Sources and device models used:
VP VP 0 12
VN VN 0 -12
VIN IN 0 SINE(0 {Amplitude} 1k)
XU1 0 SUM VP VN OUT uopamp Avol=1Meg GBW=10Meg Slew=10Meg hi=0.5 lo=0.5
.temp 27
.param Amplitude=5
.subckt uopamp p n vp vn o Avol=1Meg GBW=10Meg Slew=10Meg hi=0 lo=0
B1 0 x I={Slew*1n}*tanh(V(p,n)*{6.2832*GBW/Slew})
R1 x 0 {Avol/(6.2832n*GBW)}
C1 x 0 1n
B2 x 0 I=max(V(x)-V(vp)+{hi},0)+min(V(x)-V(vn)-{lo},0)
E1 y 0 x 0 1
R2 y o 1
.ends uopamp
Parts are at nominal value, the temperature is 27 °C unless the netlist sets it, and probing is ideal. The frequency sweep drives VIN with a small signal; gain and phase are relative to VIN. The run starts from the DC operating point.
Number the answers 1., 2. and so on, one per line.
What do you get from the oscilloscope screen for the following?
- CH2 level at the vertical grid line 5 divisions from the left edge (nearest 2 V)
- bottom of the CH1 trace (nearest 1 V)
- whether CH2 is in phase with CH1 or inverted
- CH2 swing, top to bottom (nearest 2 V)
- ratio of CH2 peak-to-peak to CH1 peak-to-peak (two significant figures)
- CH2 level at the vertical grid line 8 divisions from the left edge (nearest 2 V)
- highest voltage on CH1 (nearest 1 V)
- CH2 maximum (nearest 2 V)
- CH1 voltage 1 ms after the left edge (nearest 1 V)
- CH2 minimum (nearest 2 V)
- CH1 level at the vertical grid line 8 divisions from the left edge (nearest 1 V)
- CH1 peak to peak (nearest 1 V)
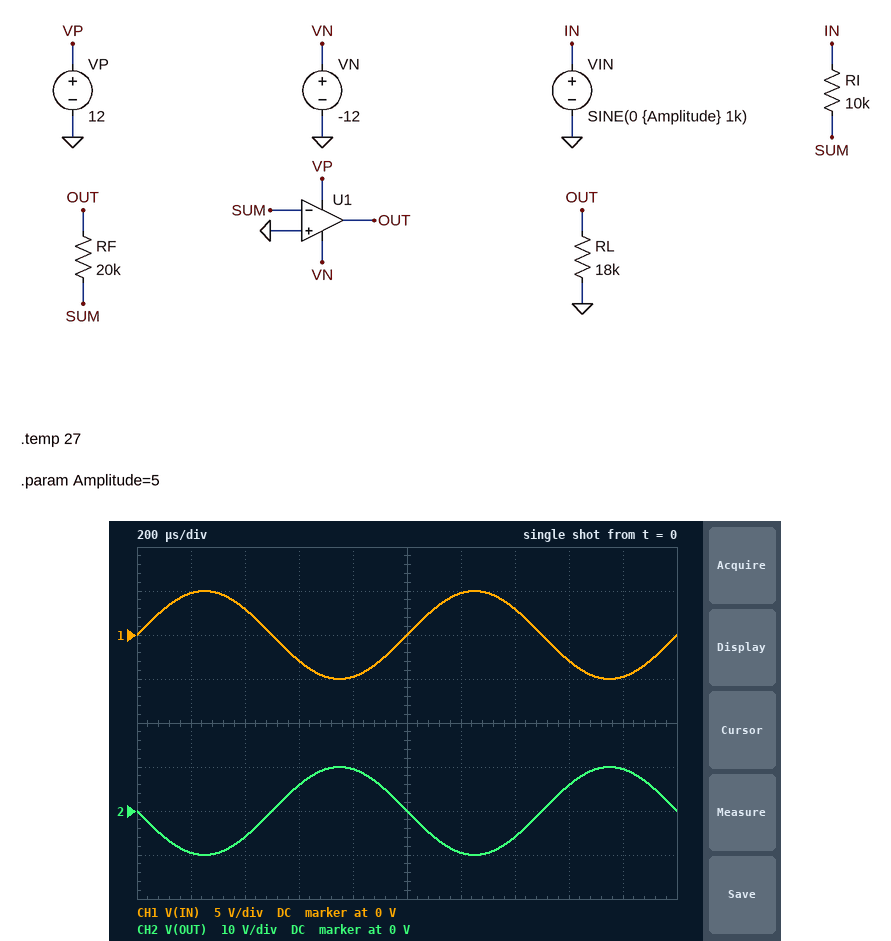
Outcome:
1. 0 V
2. -5 V
3. inverted
4. 20 V
5. 2.0
6. 6 V
7. 5 V
8. 10 V
9. 0 V
10. -10 V
11. -3 V
12. 10 V
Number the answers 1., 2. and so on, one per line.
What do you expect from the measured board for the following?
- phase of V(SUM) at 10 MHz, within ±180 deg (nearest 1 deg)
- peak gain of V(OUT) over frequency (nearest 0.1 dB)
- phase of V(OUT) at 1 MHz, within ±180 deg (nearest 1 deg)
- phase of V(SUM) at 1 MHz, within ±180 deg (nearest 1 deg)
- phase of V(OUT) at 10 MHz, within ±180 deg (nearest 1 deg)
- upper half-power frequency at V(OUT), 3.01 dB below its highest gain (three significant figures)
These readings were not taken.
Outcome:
1. 18 deg
2. 6.0 dB
3. 163 deg
4. 73 deg
5. 108 deg
6. 3.33 MHz
